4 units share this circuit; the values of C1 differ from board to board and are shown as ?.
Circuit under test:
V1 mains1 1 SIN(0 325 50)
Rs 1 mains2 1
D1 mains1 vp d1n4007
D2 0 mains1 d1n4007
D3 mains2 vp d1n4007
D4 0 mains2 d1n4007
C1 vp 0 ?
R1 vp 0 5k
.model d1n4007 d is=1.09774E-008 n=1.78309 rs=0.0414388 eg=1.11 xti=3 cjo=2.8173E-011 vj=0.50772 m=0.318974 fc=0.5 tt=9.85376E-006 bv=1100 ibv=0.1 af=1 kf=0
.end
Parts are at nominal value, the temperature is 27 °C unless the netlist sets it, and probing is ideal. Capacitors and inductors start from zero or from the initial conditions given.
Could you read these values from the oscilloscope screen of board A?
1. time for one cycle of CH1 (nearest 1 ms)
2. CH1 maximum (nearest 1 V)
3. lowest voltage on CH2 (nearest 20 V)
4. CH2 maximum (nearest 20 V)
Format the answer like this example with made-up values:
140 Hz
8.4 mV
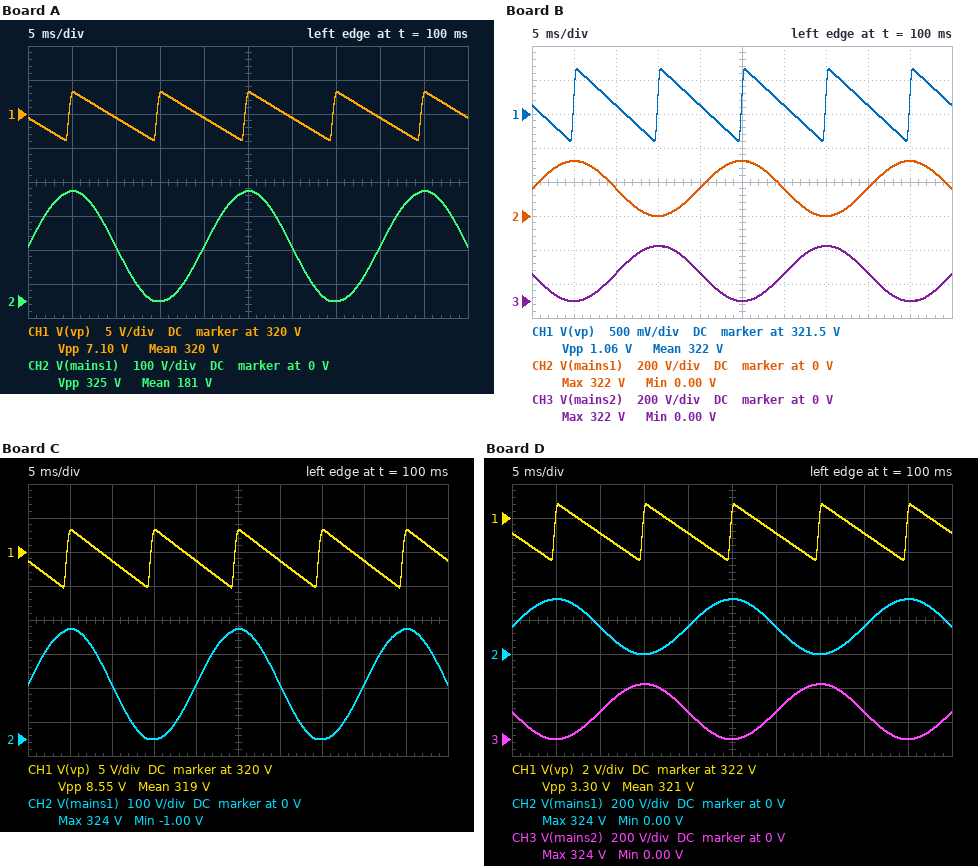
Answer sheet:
10 ms
323 V
0 V
320 V
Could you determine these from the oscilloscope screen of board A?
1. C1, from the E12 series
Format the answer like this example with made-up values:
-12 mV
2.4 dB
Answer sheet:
82 µF
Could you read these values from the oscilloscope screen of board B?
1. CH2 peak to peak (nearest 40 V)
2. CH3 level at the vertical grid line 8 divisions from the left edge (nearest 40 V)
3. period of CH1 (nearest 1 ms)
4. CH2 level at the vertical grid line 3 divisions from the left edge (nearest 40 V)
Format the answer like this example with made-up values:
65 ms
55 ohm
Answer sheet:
320 V
160 V
10 ms
0 V
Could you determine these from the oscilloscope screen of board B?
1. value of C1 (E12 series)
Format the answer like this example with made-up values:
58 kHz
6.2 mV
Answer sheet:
560 µF
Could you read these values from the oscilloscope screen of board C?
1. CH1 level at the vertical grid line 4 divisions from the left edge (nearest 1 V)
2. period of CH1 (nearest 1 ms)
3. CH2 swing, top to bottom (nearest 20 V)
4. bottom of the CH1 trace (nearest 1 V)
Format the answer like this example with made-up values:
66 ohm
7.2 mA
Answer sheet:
319 V
10 ms
320 V
315 V
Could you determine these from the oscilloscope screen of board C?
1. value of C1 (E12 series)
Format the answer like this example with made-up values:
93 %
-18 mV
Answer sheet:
68 µF
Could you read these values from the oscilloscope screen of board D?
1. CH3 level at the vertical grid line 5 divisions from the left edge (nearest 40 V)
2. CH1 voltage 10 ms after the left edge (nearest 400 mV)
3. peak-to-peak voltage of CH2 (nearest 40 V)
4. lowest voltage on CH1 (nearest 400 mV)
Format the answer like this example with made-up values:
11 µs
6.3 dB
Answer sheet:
0 V
321.2 V
320 V
319.6 V
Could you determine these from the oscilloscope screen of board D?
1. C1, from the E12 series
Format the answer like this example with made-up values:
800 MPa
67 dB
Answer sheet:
180 µF
